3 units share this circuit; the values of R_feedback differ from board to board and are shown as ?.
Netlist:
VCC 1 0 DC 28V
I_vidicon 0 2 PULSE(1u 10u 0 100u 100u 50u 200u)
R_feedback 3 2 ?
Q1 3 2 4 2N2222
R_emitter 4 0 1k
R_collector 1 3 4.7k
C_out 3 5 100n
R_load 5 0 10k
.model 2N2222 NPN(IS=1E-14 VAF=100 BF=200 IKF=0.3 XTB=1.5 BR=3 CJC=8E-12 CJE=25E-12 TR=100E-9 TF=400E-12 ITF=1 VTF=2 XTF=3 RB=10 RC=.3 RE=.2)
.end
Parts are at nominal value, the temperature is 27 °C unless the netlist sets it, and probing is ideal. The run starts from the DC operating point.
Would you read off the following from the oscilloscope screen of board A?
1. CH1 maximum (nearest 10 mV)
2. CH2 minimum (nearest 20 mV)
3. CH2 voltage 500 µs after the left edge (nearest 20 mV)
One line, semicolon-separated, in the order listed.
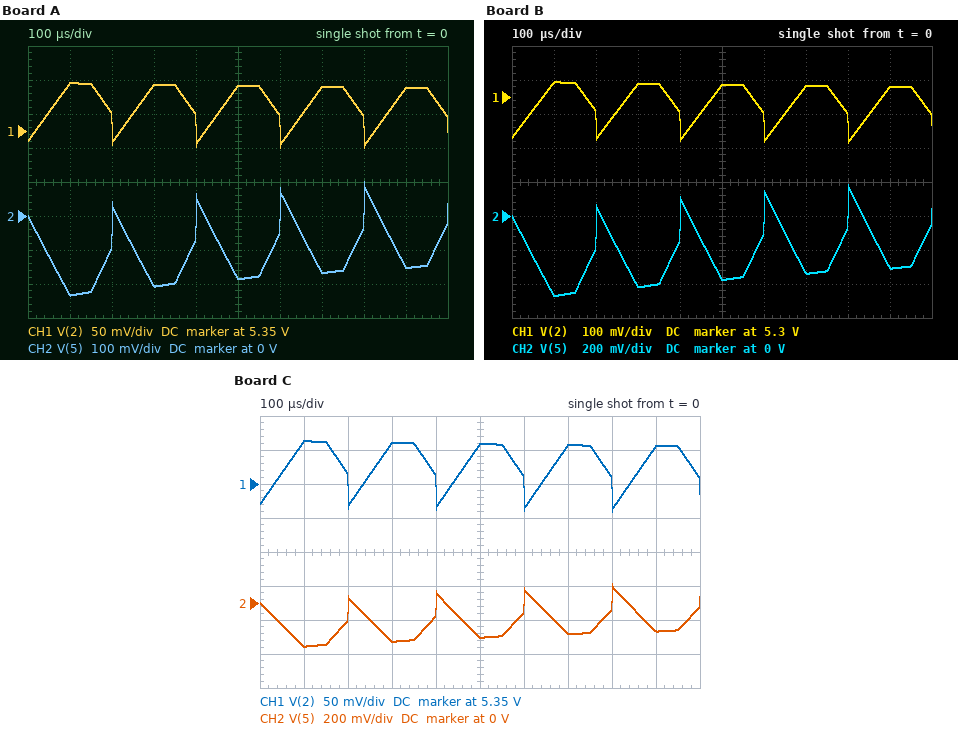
5.42 V; -240 mV; -180 mV
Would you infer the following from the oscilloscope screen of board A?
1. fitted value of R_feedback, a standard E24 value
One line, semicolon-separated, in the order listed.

39 kΩ
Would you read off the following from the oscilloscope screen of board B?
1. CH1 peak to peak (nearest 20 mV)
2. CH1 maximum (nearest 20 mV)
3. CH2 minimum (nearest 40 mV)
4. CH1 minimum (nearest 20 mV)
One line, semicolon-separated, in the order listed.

180 mV; 5.34 V; -480 mV; 5.16 V
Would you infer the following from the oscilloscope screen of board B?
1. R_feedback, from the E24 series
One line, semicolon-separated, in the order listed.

82 kΩ
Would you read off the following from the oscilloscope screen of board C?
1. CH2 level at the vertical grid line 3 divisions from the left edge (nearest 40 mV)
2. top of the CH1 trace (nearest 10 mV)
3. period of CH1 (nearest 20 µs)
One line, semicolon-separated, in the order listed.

-240 mV; 5.41 V; 200 µs
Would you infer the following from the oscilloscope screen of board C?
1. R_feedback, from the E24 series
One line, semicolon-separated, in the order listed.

43 kΩ
